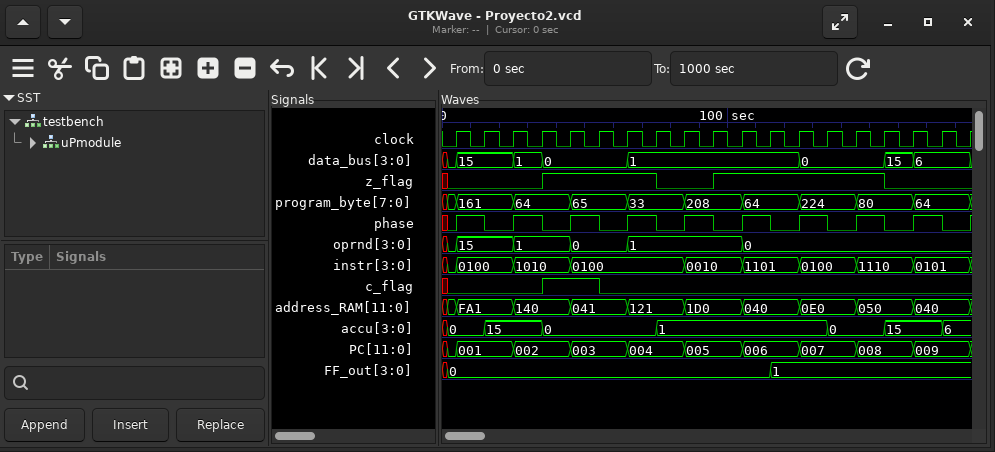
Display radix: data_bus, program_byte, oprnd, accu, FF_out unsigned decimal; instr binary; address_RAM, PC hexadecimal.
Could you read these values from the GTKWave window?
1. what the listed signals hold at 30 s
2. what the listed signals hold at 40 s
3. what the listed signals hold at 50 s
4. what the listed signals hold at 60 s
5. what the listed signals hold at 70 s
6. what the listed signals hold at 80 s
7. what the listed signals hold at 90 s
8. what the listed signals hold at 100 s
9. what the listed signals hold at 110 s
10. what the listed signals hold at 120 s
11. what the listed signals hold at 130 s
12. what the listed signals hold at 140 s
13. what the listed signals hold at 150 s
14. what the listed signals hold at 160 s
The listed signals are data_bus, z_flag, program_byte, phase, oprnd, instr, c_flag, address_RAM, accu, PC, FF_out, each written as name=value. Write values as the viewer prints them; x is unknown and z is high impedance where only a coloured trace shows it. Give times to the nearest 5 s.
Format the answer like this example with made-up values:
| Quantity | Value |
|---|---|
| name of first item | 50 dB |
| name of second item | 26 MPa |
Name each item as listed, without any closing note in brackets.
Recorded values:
| Quantity | Value |
|---|---|
| what the listed signals hold at 30 s | data_bus=1, z_flag=0, program_byte=64, phase=1, oprnd=1, instr=1010, c_flag=0, address_RAM=140, accu=15, PC=002, FF_out=0 |
| what the listed signals hold at 40 s | data_bus=0, z_flag=1, program_byte=64, phase=0, oprnd=1, instr=1010, c_flag=1, address_RAM=140, accu=0, PC=002, FF_out=0 |
| what the listed signals hold at 50 s | data_bus=0, z_flag=1, program_byte=65, phase=1, oprnd=0, instr=0100, c_flag=1, address_RAM=041, accu=0, PC=003, FF_out=0 |
| what the listed signals hold at 60 s | data_bus=0, z_flag=1, program_byte=65, phase=0, oprnd=0, instr=0100, c_flag=0, address_RAM=041, accu=0, PC=003, FF_out=0 |
| what the listed signals hold at 70 s | data_bus=1, z_flag=1, program_byte=33, phase=1, oprnd=1, instr=0100, c_flag=0, address_RAM=121, accu=0, PC=004, FF_out=0 |
| what the listed signals hold at 80 s | data_bus=1, z_flag=0, program_byte=33, phase=0, oprnd=1, instr=0100, c_flag=0, address_RAM=121, accu=1, PC=004, FF_out=0 |
| what the listed signals hold at 90 s | data_bus=1, z_flag=0, program_byte=208, phase=1, oprnd=1, instr=0010, c_flag=0, address_RAM=1D0, accu=1, PC=005, FF_out=0 |
| what the listed signals hold at 100 s | data_bus=1, z_flag=1, program_byte=208, phase=0, oprnd=1, instr=0010, c_flag=0, address_RAM=1D0, accu=1, PC=005, FF_out=0 |
| what the listed signals hold at 110 s | data_bus=1, z_flag=1, program_byte=64, phase=1, oprnd=0, instr=1101, c_flag=0, address_RAM=040, accu=1, PC=006, FF_out=0 |
| what the listed signals hold at 120 s | data_bus=1, z_flag=1, program_byte=64, phase=0, oprnd=0, instr=1101, c_flag=0, address_RAM=040, accu=1, PC=006, FF_out=1 |
| what the listed signals hold at 130 s | data_bus=0, z_flag=1, program_byte=224, phase=1, oprnd=0, instr=0100, c_flag=0, address_RAM=0E0, accu=1, PC=007, FF_out=1 |
| what the listed signals hold at 140 s | data_bus=0, z_flag=1, program_byte=224, phase=0, oprnd=0, instr=0100, c_flag=0, address_RAM=0E0, accu=0, PC=007, FF_out=1 |
| what the listed signals hold at 150 s | data_bus=0, z_flag=1, program_byte=80, phase=1, oprnd=0, instr=1110, c_flag=0, address_RAM=050, accu=0, PC=008, FF_out=1 |
| what the listed signals hold at 160 s | data_bus=15, z_flag=0, program_byte=80, phase=0, oprnd=0, instr=1110, c_flag=0, address_RAM=050, accu=15, PC=008, FF_out=1 |
